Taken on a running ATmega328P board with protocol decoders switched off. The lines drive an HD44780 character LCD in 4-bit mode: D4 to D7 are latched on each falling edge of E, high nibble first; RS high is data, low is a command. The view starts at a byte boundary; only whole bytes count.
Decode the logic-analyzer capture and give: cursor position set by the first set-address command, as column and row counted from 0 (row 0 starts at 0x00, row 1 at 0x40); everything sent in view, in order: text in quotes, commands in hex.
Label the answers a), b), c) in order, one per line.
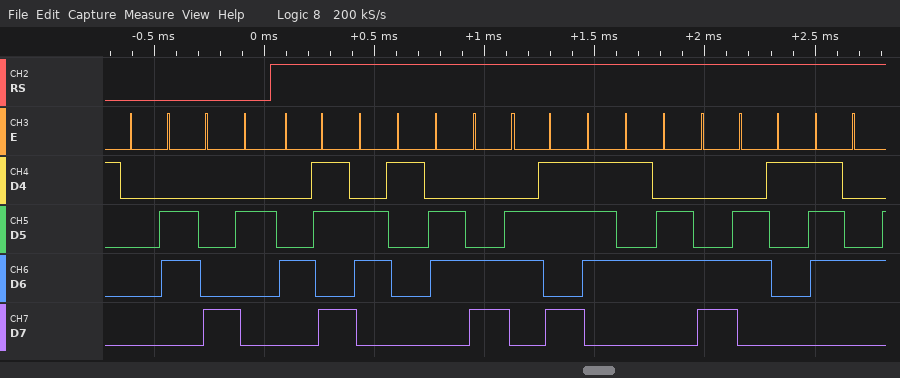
a) column 2, row 0
b) 0x06 0x82 "Kalkulat"
